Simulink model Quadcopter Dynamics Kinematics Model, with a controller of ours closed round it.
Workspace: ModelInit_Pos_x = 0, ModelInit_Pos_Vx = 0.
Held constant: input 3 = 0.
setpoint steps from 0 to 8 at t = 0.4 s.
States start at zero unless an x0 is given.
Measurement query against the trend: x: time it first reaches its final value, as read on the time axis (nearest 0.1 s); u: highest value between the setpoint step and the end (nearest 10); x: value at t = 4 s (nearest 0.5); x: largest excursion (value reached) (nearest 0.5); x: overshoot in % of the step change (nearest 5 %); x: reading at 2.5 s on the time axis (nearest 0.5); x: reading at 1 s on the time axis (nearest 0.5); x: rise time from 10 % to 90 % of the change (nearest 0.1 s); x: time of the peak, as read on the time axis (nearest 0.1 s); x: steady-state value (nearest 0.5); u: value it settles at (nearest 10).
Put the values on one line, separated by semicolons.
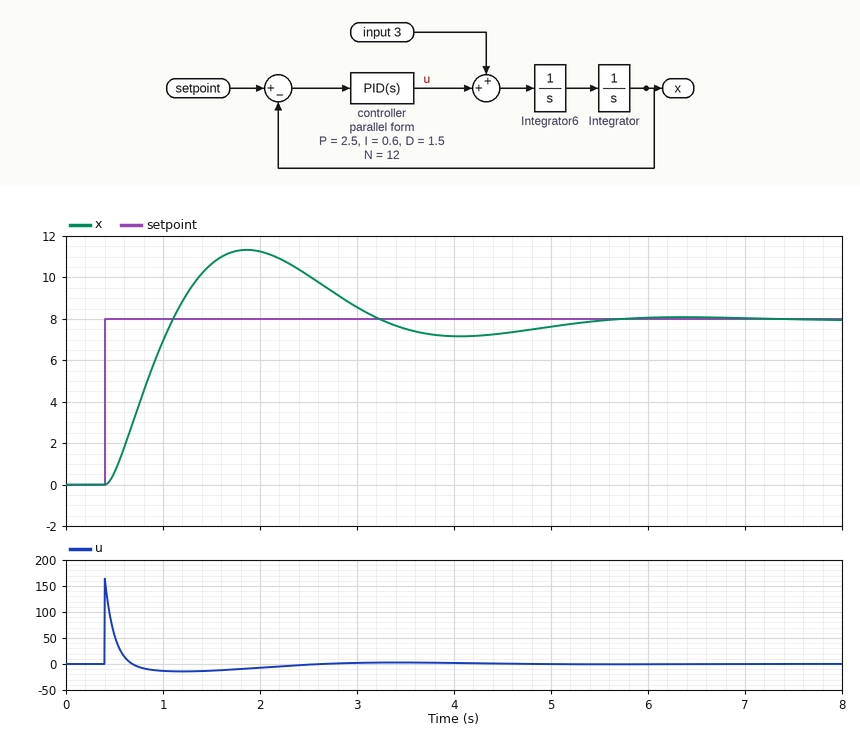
1.1 s; 160; 7.0; 11.5; 40 %; 10.0; 7.0; 0.5 s; 1.9 s; 8.0; 0
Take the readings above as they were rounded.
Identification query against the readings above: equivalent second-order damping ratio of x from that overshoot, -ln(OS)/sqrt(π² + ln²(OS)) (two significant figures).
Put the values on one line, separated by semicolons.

0.28
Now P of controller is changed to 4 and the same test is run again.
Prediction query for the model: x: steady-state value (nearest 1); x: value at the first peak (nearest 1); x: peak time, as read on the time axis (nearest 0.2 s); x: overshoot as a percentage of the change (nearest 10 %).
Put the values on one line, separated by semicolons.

8; 12; 1.6 s; 50 %
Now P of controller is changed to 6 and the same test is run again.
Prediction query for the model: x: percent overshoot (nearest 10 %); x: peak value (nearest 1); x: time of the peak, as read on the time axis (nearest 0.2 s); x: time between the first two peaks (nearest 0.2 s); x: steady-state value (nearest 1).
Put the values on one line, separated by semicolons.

50 %; 12; 1.4 s; 2.6 s; 8
